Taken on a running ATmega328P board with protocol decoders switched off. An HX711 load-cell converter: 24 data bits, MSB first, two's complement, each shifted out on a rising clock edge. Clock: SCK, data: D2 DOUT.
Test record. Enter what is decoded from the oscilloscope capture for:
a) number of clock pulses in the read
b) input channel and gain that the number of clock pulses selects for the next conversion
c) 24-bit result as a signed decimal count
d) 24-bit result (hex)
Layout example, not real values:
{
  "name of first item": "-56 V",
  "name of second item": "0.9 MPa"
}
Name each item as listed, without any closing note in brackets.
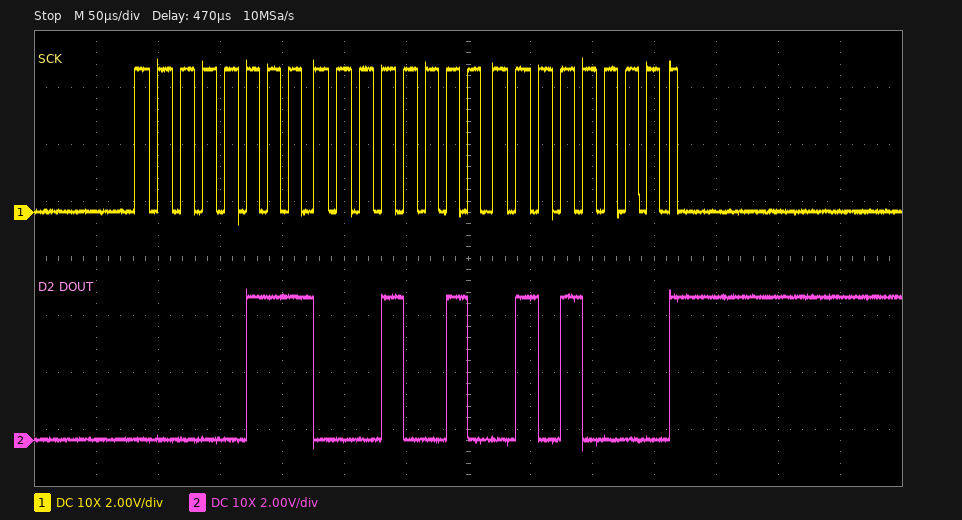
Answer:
{
  "number of clock pulses in the read": "25",
  "input channel and gain that the number of clock pulses selects for the next conversion": "channel A, gain 128",
  "24-bit result as a signed decimal count": "463440",
  "24-bit result": "0x071250"
}
